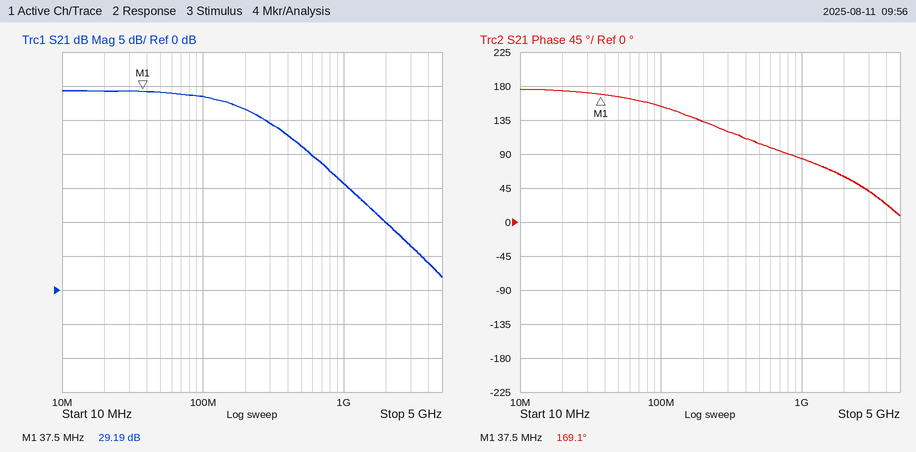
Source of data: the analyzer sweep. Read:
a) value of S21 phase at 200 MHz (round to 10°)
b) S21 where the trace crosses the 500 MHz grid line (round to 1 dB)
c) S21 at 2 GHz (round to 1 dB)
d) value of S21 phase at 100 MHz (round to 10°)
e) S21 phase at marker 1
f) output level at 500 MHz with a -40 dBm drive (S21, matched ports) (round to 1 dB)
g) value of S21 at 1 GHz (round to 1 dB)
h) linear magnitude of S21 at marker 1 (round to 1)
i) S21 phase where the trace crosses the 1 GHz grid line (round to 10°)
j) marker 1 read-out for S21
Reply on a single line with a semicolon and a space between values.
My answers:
130°; 21 dB; 10 dB; 150°; 169.1°; -19 dBm; 16 dB; 29; 80°; 29.19 dB
